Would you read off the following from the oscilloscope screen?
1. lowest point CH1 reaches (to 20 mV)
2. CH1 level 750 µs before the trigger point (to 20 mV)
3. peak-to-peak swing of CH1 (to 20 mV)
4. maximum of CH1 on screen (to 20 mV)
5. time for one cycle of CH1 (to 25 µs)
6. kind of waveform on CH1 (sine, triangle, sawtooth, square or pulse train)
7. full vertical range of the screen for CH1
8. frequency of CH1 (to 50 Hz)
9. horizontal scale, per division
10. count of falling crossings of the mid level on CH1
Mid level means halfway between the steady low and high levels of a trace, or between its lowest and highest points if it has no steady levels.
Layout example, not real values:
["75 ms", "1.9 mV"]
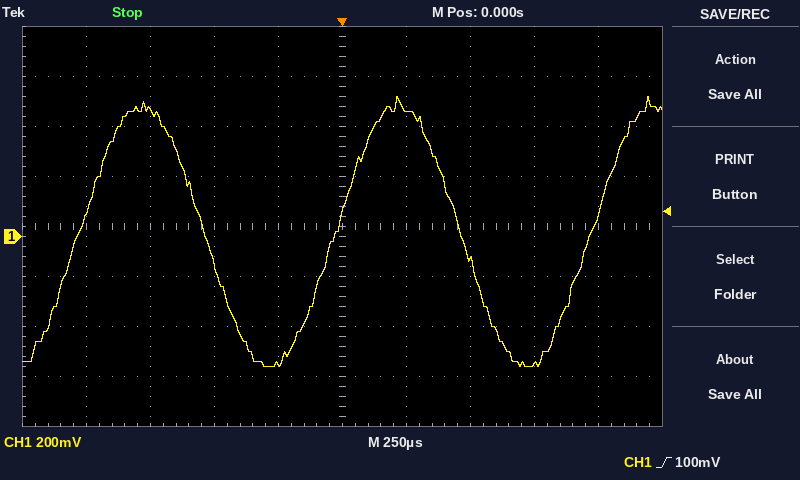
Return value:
["-520 mV", "500 mV", "1.08 V", "560 mV", "1.000 ms", "sine", "1.6 V", "1.00 kHz", "250 µs", "2"]
